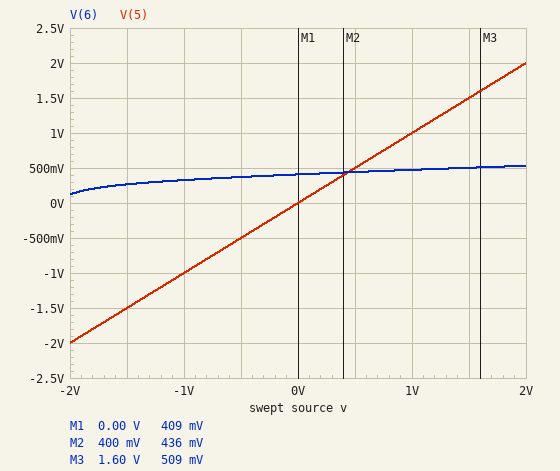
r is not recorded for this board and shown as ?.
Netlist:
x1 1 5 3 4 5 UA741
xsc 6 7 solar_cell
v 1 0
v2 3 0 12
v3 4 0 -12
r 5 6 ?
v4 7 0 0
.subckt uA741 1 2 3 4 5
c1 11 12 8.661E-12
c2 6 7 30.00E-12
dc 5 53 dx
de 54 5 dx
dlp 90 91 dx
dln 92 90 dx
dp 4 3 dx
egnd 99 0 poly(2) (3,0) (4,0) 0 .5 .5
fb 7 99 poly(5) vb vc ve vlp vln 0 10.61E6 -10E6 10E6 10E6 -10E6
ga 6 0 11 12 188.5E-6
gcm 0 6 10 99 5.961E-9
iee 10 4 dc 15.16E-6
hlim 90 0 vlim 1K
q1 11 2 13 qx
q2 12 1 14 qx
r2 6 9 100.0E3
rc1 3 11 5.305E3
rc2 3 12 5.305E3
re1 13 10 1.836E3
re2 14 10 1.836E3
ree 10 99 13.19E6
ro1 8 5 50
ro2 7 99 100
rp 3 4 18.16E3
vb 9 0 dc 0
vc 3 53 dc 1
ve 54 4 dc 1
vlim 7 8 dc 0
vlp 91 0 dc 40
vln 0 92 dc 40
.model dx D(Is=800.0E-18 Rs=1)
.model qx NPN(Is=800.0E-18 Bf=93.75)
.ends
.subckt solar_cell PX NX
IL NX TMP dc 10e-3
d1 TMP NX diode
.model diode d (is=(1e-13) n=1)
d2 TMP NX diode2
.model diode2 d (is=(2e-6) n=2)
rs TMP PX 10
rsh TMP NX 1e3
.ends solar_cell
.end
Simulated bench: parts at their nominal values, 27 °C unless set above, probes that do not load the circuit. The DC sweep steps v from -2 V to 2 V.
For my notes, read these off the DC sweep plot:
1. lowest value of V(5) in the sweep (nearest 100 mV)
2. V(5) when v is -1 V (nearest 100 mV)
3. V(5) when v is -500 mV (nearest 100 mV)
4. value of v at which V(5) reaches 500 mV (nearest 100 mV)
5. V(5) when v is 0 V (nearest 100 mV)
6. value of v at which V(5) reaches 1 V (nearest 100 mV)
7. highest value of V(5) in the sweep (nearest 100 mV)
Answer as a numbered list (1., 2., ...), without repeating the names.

1. -2.0 V
2. -1.0 V
3. -500 mV
4. 500 mV
5. 0 V
6. 1.0 V
7. 2.0 V
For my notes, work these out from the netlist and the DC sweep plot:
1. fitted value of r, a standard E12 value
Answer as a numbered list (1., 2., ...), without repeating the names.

1. 220 Ω
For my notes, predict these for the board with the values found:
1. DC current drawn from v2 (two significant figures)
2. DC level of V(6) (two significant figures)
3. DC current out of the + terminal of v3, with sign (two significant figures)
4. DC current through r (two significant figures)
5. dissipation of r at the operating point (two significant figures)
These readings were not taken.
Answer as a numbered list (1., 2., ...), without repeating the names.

1. 1.3 mA
2. 410 mV
3. -1.3 mA
4. 1.9 mA
5. 760 µW
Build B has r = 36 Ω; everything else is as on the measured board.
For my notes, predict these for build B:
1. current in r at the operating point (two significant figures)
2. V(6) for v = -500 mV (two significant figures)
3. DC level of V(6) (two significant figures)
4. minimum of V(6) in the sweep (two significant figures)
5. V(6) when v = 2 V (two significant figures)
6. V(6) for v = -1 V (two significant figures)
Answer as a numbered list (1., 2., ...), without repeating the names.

1. 7.7 mA
2. -140 mV
3. 280 mV
4. -1.6 V
5. 840 mV
6. -620 mV
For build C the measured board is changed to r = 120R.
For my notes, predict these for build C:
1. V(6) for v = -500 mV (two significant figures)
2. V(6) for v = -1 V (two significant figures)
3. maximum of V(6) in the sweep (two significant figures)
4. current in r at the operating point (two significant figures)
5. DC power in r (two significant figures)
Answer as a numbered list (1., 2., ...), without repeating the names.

1. 310 mV
2. 150 mV
3. 600 mV
4. 3.2 mA
5. 1.2 mW
